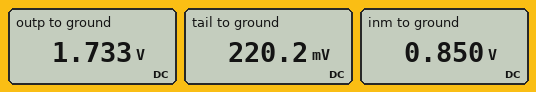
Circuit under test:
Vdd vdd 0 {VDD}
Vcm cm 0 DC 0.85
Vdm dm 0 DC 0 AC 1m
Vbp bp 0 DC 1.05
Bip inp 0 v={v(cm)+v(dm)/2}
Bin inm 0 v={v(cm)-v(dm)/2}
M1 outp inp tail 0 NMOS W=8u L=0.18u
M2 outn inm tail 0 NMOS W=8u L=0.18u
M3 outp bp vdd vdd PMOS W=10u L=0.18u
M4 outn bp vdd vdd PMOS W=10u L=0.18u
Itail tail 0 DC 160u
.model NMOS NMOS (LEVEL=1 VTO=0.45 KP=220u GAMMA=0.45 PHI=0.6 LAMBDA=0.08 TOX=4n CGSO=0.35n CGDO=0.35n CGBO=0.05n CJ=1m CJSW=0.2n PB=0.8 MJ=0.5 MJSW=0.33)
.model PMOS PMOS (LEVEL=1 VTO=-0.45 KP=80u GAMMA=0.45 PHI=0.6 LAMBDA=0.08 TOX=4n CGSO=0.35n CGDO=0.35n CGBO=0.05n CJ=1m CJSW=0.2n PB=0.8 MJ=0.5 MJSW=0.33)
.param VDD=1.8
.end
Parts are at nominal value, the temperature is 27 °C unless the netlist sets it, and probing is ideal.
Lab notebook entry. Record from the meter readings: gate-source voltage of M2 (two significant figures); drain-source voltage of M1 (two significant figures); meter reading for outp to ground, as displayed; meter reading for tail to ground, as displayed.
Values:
630 mV
1.5 V
1.733 V
220.2 mV
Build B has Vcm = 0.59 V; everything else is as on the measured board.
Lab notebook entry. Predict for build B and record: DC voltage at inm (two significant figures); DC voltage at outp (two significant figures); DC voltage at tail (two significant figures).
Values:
590 mV
1.7 V
16 mV
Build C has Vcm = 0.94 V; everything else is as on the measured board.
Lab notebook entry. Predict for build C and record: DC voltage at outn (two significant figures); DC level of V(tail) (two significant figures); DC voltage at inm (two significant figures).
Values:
1.7 V
290 mV
940 mV
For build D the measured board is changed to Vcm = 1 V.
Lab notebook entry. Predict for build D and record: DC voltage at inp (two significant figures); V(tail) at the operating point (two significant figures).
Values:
1.0 V
340 mV
